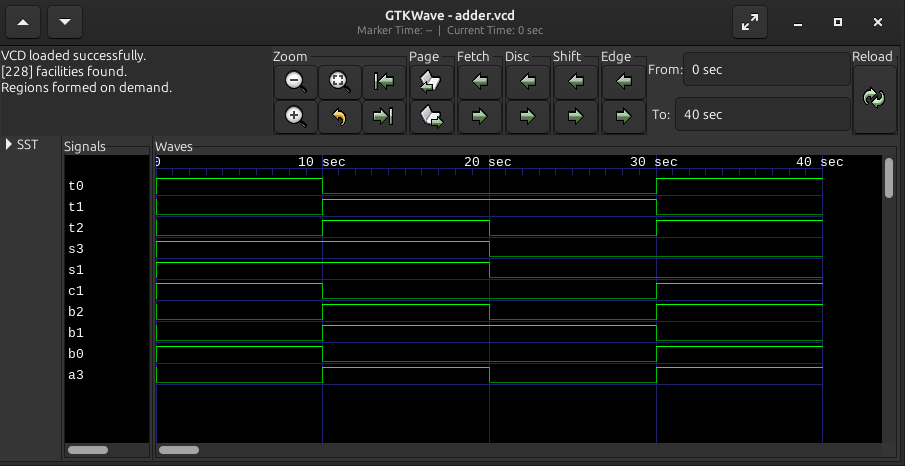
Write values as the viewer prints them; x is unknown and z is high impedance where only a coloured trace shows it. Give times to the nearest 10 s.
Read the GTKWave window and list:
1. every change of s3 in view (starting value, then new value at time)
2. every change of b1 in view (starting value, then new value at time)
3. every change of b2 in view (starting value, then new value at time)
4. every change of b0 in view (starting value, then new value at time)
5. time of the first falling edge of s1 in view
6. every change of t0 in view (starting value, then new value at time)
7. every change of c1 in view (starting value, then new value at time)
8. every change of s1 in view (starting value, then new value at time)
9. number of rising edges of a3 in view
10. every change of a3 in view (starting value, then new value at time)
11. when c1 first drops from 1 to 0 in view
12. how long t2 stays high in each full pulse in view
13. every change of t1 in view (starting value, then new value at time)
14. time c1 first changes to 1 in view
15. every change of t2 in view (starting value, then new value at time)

1, 0 at 20 s
0, 1 at 10 s, 0 at 30 s
0, 1 at 10 s, 0 at 20 s, 1 at 30 s
1, 0 at 10 s, 1 at 30 s
20 s
1, 0 at 10 s, 1 at 30 s
1, 0 at 10 s, 1 at 30 s
1, 0 at 20 s
2
0, 1 at 10 s, 0 at 20 s, 1 at 30 s
10 s
10 s
0, 1 at 10 s, 0 at 30 s
30 s
0, 1 at 10 s, 0 at 20 s, 1 at 30 s
